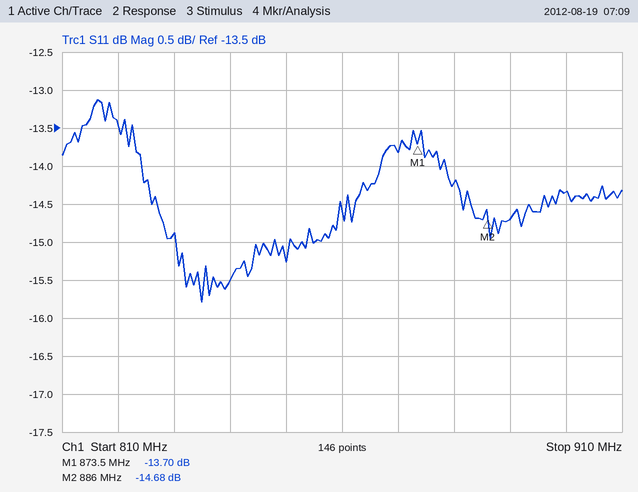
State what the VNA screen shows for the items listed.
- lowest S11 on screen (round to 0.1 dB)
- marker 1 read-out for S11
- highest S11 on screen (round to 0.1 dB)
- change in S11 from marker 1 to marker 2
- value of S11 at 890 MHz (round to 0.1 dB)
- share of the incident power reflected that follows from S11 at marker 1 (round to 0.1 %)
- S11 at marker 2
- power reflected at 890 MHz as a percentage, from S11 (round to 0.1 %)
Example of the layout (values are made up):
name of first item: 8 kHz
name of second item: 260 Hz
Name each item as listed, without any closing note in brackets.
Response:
lowest S11 on screen: -15.8 dB
marker 1 read-out for S11: -13.70 dB
highest S11 on screen: -13.1 dB
change in S11 from marker 1 to marker 2: -0.98 dB
value of S11 at 890 MHz: -14.7 dB
share of the incident power reflected that follows from S11 at marker 1: 4.3 %
S11 at marker 2: -14.68 dB
power reflected at 890 MHz as a percentage, from S11: 3.4 %
